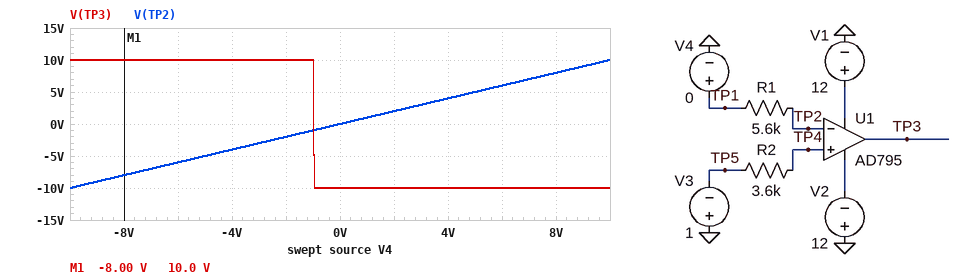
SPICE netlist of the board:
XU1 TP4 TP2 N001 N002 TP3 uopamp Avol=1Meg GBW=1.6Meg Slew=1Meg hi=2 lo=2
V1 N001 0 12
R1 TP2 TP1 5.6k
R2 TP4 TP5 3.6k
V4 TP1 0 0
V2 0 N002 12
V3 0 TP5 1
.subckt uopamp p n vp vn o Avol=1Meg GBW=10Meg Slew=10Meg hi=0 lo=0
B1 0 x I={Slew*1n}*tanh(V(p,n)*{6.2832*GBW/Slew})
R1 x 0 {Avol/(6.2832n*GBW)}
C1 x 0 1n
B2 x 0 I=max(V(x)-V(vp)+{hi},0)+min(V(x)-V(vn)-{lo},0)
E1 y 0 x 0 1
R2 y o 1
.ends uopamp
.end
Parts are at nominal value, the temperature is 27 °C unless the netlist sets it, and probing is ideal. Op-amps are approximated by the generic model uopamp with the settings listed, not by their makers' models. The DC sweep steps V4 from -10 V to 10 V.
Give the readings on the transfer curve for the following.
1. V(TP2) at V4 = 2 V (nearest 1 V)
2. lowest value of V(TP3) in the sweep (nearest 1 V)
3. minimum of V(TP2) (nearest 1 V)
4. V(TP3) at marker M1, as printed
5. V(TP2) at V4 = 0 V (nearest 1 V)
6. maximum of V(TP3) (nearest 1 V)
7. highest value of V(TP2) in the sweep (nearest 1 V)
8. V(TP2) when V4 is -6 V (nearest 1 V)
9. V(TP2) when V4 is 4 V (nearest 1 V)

2 V
-10 V
-10 V
10.0 V
0 V
10 V
10 V
-6 V
4 V
